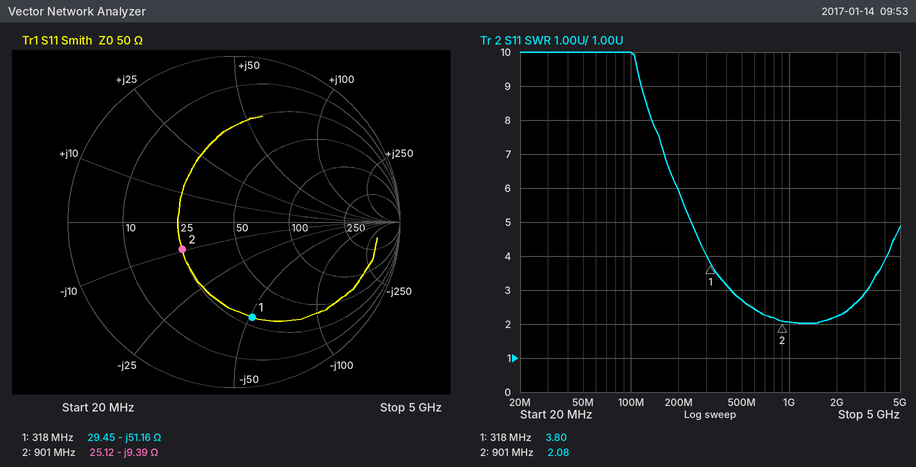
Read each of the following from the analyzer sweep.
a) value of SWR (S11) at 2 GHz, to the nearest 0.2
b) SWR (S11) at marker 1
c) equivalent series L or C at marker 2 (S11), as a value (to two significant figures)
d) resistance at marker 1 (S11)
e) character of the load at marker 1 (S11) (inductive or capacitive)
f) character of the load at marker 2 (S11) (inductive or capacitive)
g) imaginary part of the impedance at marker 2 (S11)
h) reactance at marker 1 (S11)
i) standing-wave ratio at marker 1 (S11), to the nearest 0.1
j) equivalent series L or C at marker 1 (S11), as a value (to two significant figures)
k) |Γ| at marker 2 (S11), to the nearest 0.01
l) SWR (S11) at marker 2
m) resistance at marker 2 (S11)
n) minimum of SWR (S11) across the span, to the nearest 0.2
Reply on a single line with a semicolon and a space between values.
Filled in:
2.2; 3.80; 19 pF; 29.45 Ω; capacitive; capacitive; -9.39 Ω; -51.16 Ω; 3.8; 9.8 pF; 0.35; 2.08; 25.12 Ω; 2.0
